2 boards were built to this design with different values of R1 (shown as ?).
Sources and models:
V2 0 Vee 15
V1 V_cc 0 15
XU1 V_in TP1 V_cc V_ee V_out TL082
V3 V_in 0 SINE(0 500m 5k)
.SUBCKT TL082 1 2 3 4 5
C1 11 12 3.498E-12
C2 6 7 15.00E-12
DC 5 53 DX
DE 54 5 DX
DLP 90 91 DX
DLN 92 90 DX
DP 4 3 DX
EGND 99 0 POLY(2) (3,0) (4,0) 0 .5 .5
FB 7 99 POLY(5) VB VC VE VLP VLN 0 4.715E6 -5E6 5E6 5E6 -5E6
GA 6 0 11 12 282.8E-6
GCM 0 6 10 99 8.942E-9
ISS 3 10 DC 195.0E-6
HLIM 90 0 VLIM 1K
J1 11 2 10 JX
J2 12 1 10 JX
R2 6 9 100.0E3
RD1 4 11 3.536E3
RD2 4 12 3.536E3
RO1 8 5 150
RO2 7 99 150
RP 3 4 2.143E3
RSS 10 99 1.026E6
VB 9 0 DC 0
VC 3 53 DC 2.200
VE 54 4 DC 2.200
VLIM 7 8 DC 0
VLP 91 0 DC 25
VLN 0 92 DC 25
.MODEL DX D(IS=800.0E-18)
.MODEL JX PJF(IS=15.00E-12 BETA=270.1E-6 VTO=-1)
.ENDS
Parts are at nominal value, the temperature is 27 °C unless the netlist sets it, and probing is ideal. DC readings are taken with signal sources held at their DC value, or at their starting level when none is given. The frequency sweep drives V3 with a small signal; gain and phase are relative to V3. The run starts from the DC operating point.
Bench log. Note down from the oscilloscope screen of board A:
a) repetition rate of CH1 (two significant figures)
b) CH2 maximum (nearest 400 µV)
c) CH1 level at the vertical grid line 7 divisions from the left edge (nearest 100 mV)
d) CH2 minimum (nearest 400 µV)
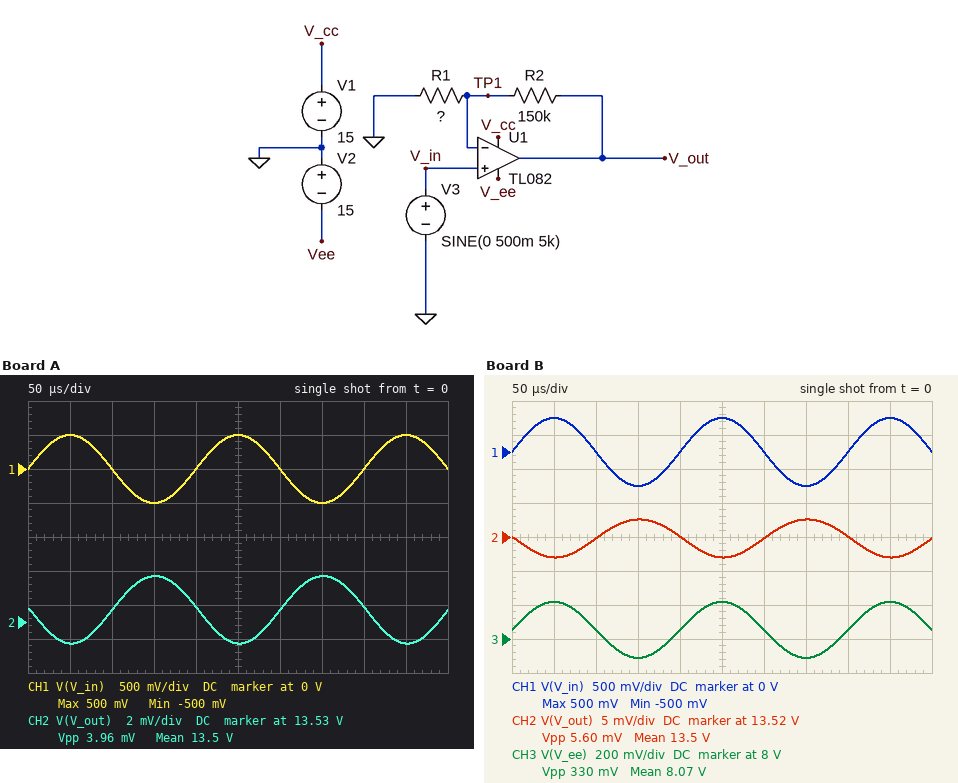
5.0 kHz
13.5288 V
-500 mV
13.5248 V
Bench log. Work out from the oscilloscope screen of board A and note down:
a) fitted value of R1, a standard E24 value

13 kΩ
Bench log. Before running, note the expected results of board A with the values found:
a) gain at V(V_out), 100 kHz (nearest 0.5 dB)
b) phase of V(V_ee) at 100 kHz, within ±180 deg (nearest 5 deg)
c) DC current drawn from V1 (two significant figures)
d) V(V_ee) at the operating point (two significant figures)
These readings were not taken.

-51.0 dB
0 deg
2.0 mA
8.4 V
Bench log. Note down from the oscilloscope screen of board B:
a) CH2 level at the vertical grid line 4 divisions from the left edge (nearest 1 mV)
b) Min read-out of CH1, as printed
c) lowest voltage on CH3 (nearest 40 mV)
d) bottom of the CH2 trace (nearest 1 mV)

13.520 V
-500 mV
7.88 V
13.517 V
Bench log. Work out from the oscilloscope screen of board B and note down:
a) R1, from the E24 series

6.2 kΩ
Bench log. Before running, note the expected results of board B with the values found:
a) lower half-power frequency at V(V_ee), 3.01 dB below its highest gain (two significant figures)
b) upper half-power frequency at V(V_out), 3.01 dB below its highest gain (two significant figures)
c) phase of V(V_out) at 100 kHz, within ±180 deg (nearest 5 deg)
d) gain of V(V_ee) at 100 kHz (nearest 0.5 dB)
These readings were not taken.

8.9 MHz
110 kHz
135 deg
-9.5 dB
